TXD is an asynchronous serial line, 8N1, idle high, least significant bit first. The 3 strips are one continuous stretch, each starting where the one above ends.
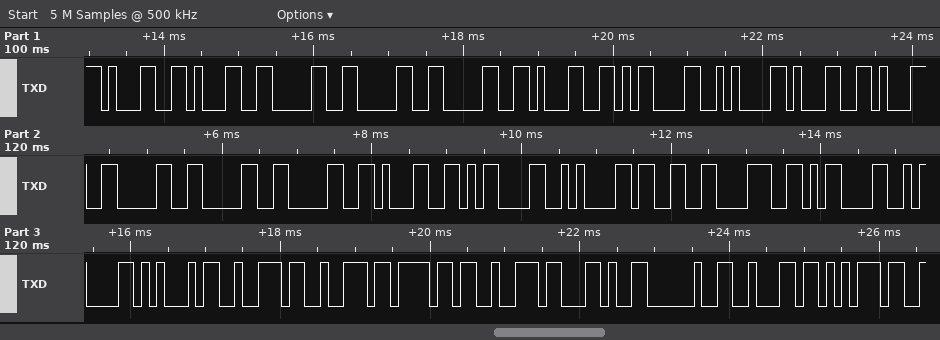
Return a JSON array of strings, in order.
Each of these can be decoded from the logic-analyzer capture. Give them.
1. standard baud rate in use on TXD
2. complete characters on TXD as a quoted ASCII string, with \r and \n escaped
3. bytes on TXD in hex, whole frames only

["9600 baud", "\"110001\\r\\n110001\\r\\n38\\r\\nError, bu\"", "31 31 30 30 30 31 0D 0A 31 31 30 30 30 31 0D 0A 33 38 0D 0A 45 72 72 6F 72 2C 20 62 75"]
